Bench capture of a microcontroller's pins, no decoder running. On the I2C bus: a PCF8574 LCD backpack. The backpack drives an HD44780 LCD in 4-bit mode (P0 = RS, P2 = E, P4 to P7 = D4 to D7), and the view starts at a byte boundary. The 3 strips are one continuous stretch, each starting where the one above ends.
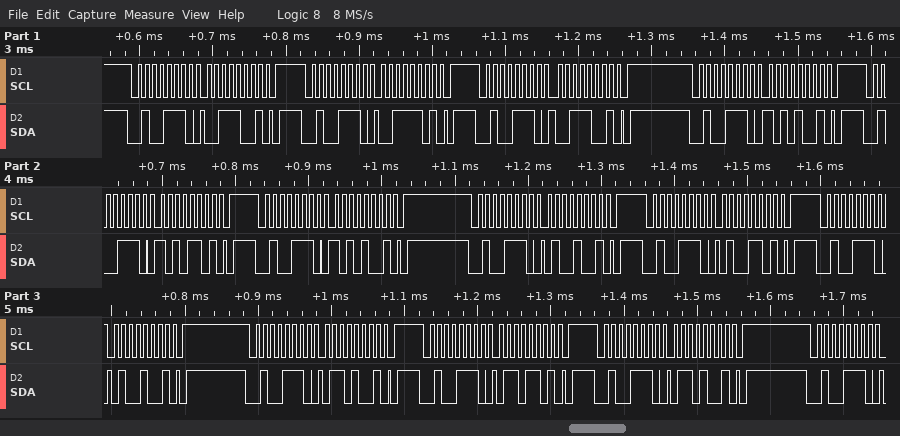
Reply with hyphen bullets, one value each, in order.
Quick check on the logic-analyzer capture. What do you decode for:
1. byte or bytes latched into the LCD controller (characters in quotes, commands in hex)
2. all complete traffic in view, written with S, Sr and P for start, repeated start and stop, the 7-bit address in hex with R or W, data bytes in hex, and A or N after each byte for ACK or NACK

- ':' 'F'
- S 27W A 39 A P S 27W A 3D A P S 27W A 39 A P S 27W A A9 A P S 27W A AD A P S 27W A A9 A P S 27W A 49 A P S 27W A 4D A P S 27W A 49 A P S 27W A 69 A P S 27W A 6D A P S 27W A 69 A P S 27W A
